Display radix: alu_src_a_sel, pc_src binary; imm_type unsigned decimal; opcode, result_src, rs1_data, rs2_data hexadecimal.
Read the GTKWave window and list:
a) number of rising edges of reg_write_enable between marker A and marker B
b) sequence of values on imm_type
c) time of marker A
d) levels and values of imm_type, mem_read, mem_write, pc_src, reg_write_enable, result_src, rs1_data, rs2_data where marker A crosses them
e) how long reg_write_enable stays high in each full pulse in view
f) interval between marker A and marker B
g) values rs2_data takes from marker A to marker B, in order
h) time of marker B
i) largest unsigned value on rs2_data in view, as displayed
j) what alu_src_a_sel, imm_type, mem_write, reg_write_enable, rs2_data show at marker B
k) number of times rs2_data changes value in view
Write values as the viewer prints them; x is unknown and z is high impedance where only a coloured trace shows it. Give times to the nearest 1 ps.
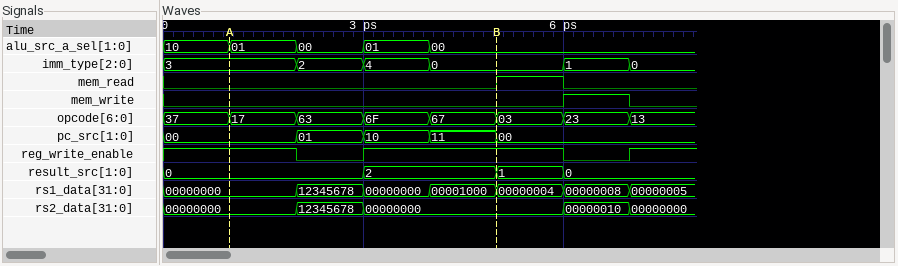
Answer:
1
3, 2, 4, 0, 1, 0
1 ps
imm_type=3, mem_read=0, mem_write=0, pc_src=00, reg_write_enable=1, result_src=0, rs1_data=00000000, rs2_data=00000000
3 ps
4 ps
00000000, 12345678, 00000000
5 ps
12345678
alu_src_a_sel=00, imm_type=0, mem_write=0, reg_write_enable=1, rs2_data=00000000
4
